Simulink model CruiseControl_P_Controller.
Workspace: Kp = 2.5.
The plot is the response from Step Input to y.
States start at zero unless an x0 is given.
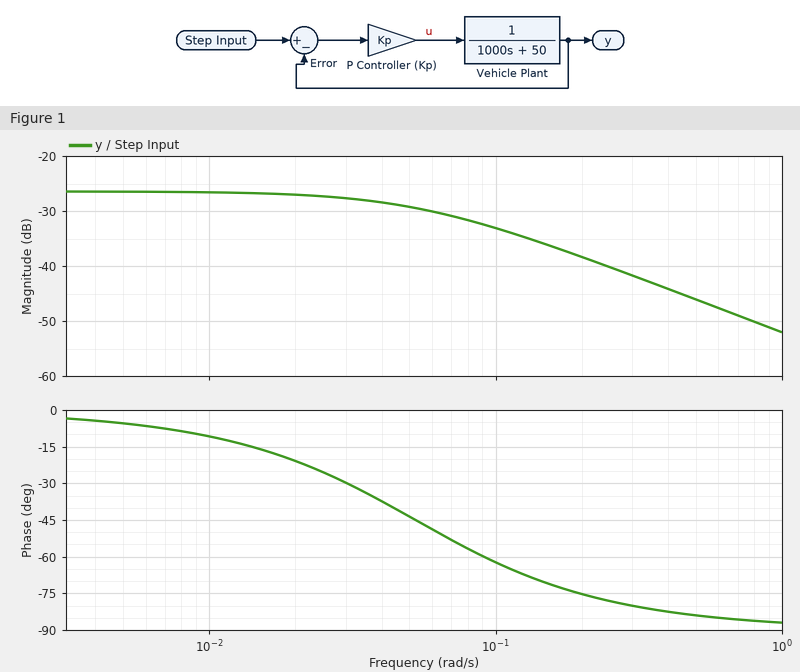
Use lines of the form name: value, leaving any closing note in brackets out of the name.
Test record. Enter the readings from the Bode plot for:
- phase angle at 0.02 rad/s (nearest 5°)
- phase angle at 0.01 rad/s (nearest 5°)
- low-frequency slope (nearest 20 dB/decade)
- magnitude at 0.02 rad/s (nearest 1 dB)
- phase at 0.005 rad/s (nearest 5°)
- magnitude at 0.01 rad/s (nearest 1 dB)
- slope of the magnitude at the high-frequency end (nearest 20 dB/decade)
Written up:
phase angle at 0.02 rad/s: -20°
phase angle at 0.01 rad/s: -10°
low-frequency slope: 0 dB/decade
magnitude at 0.02 rad/s: -27 dB
phase at 0.005 rad/s: -5°
magnitude at 0.01 rad/s: -27 dB
slope of the magnitude at the high-frequency end: -20 dB/decade
